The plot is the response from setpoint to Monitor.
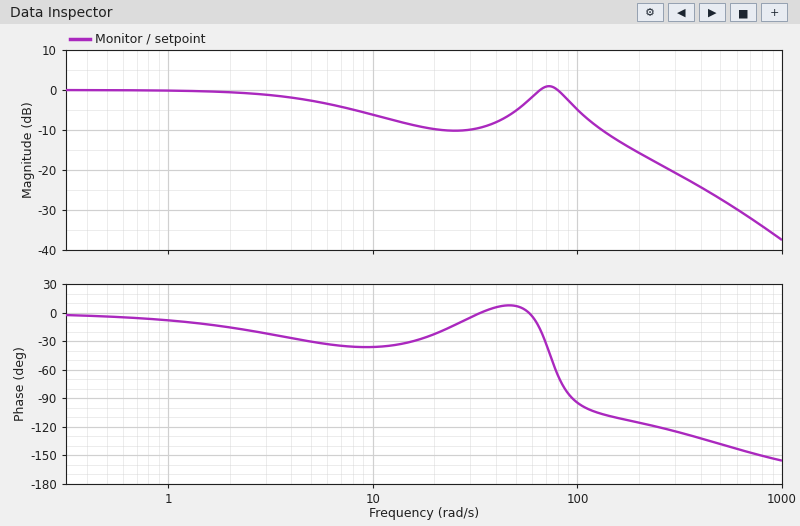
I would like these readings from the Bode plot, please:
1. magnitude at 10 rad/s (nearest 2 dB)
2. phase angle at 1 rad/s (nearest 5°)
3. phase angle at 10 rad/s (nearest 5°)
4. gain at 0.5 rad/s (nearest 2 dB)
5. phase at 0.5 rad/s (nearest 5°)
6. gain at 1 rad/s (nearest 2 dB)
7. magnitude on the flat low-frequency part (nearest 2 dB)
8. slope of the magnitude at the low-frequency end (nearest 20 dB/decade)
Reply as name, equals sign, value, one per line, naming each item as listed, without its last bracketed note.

magnitude at 10 rad/s = -6 dB
phase angle at 1 rad/s = -10°
phase angle at 10 rad/s = -35°
gain at 0.5 rad/s = 0 dB
phase at 0.5 rad/s = -5°
gain at 1 rad/s = 0 dB
magnitude on the flat low-frequency part = 0 dB
slope of the magnitude at the low-frequency end = 0 dB/decade
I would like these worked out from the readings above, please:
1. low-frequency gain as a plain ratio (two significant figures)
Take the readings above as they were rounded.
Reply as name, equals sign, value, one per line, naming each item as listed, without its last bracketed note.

low-frequency gain as a plain ratio = 1.0
